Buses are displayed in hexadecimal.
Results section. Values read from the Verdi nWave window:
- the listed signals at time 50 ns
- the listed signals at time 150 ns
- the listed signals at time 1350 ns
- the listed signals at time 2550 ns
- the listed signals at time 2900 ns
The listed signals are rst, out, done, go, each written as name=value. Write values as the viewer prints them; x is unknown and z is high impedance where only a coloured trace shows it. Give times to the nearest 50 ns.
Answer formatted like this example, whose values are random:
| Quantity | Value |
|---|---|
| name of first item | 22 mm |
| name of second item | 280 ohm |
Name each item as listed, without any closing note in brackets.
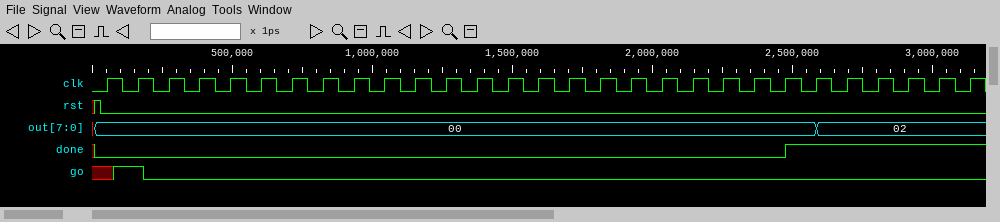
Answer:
| Quantity | Value |
|---|---|
| the listed signals at time 50 ns | rst=0, out=00, done=0, go=x |
| the listed signals at time 150 ns | rst=0, out=00, done=0, go=1 |
| the listed signals at time 1350 ns | rst=0, out=00, done=0, go=0 |
| the listed signals at time 2550 ns | rst=0, out=00, done=1, go=0 |
| the listed signals at time 2900 ns | rst=0, out=02, done=1, go=0 |
